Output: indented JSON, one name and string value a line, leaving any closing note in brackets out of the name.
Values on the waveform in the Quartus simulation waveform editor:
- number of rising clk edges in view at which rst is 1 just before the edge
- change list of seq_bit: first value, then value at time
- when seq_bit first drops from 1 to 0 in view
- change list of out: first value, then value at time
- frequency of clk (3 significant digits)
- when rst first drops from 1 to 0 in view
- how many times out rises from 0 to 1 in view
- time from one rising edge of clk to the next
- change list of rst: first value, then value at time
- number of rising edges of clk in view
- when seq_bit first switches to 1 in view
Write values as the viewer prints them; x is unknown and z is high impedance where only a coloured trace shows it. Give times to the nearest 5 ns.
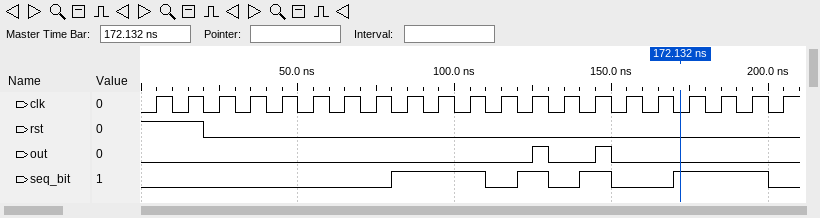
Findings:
{
  "number of rising clk edges in view at which rst is 1 just before the edge": "2",
  "change list of seq_bit: first value, then value at time": "0, 1 at 80 ns, 0 at 110 ns, 1 at 120 ns, 0 at 130 ns, 1 at 140 ns, 0 at 150 ns, 1 at 170 ns, 0 at 200 ns",
  "when seq_bit first drops from 1 to 0 in view": "110 ns",
  "change list of out: first value, then value at time": "0, 1 at 125 ns, 0 at 130 ns, 1 at 145 ns, 0 at 150 ns",
  "frequency of clk": "100 MHz",
  "when rst first drops from 1 to 0 in view": "20 ns",
  "how many times out rises from 0 to 1 in view": "2",
  "time from one rising edge of clk to the next": "10 ns",
  "change list of rst: first value, then value at time": "1, 0 at 20 ns",
  "number of rising edges of clk in view": "21",
  "when seq_bit first switches to 1 in view": "80 ns"
}
